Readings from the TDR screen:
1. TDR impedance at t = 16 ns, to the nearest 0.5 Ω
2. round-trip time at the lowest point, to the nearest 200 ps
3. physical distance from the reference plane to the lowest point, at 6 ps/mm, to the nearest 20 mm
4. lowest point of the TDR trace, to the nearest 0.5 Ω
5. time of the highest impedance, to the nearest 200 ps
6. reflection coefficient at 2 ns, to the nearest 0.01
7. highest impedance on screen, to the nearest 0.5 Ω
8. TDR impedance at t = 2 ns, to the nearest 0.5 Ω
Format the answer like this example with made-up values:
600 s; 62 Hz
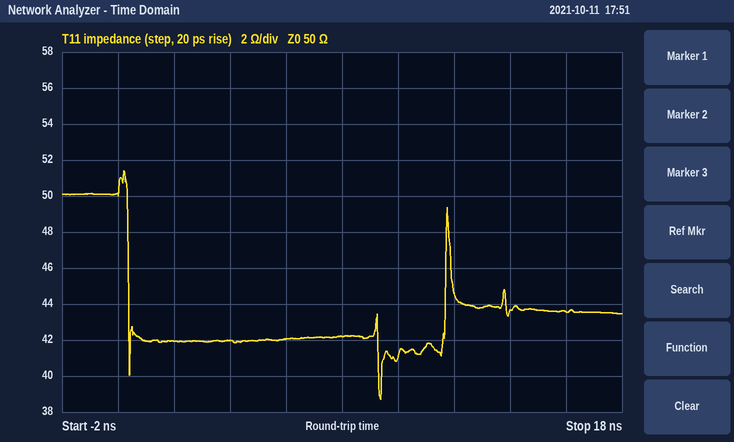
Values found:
43.5 Ω; 9.4 ns; 780 mm; 38.5 Ω; 200 ps; -0.09; 51.5 Ω; 42.0 Ω
